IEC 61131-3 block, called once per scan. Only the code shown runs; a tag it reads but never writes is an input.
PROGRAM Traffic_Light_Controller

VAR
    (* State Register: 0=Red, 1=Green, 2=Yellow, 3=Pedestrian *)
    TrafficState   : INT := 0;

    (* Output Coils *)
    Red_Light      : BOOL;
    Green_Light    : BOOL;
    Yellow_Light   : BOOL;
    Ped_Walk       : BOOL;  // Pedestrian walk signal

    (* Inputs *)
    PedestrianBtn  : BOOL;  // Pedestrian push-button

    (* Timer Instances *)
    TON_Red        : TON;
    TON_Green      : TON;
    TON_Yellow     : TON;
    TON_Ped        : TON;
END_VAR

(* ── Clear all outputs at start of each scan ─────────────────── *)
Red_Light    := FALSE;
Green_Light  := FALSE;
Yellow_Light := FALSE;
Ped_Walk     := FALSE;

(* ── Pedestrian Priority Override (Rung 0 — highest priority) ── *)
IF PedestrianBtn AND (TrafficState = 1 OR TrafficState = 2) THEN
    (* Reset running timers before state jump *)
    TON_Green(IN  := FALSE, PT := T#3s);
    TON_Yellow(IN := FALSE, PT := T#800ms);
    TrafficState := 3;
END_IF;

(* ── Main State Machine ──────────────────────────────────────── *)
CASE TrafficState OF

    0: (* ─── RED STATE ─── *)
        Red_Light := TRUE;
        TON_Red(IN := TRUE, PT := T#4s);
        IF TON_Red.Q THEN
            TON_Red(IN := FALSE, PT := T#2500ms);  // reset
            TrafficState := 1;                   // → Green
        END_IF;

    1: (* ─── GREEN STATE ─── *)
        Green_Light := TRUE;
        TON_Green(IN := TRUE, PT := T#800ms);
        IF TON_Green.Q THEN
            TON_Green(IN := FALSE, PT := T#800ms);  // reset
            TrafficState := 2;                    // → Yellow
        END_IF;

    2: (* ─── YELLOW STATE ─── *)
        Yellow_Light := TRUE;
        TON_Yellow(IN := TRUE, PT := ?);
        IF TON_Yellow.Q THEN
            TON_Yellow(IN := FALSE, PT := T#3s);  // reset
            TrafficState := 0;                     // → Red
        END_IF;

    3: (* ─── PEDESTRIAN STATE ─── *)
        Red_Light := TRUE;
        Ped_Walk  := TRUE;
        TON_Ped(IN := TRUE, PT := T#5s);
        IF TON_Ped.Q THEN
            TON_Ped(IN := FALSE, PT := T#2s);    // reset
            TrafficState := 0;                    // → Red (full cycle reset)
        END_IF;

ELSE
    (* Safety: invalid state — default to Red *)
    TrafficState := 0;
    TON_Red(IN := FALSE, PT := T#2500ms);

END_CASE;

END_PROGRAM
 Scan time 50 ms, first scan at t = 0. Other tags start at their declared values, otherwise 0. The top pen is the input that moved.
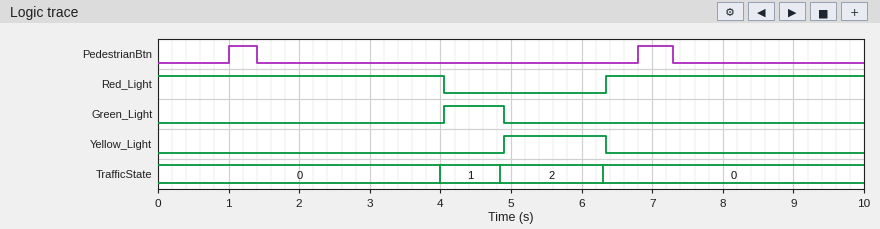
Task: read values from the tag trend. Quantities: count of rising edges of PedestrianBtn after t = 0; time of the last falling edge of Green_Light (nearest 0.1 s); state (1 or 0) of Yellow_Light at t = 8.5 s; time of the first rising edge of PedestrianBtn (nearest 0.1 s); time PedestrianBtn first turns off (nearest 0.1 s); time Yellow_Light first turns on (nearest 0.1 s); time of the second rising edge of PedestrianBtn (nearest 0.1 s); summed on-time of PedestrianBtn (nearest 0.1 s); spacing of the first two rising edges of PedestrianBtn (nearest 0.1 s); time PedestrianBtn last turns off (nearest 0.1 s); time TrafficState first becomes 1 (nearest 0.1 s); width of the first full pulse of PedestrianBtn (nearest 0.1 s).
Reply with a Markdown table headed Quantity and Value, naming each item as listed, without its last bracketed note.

| Quantity | Value |
|---|---|
| count of rising edges of PedestrianBtn after t = 0 | 2 |
| time of the last falling edge of Green_Light | 4.9 s |
| state (1 or 0) of Yellow_Light at t = 8.5 s | 0 |
| time of the first rising edge of PedestrianBtn | 1.0 s |
| time PedestrianBtn first turns off | 1.4 s |
| time Yellow_Light first turns on | 4.9 s |
| time of the second rising edge of PedestrianBtn | 6.8 s |
| summed on-time of PedestrianBtn | 0.9 s |
| spacing of the first two rising edges of PedestrianBtn | 5.8 s |
| time PedestrianBtn last turns off | 7.3 s |
| time TrafficState first becomes 1 | 4.0 s |
| width of the first full pulse of PedestrianBtn | 0.4 s |
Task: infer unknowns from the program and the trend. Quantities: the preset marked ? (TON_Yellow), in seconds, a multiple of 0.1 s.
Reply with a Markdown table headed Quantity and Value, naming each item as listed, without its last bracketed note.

| Quantity | Value |
|---|---|
| the preset marked ? (TON_Yellow), in seconds, a multiple of 0.1 s | 1.4 s |
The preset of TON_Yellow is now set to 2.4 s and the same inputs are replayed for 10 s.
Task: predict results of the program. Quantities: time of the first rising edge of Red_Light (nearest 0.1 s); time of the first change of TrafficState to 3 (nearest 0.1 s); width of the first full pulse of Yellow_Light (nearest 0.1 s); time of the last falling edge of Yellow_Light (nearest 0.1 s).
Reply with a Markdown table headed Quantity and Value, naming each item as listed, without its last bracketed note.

| Quantity | Value |
|---|---|
| time of the first rising edge of Red_Light | 6.8 s |
| time of the first change of TrafficState to 3 | 6.8 s |
| width of the first full pulse of Yellow_Light | 1.9 s |
| time of the last falling edge of Yellow_Light | 6.8 s |
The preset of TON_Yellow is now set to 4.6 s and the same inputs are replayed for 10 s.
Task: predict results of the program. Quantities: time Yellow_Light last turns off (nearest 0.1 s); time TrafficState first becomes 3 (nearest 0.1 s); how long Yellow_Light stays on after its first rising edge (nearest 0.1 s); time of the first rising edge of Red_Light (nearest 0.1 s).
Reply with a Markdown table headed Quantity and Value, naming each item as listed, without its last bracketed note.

| Quantity | Value |
|---|---|
| time Yellow_Light last turns off | 6.8 s |
| time TrafficState first becomes 3 | 6.8 s |
| how long Yellow_Light stays on after its first rising edge | 1.9 s |
| time of the first rising edge of Red_Light | 6.8 s |
